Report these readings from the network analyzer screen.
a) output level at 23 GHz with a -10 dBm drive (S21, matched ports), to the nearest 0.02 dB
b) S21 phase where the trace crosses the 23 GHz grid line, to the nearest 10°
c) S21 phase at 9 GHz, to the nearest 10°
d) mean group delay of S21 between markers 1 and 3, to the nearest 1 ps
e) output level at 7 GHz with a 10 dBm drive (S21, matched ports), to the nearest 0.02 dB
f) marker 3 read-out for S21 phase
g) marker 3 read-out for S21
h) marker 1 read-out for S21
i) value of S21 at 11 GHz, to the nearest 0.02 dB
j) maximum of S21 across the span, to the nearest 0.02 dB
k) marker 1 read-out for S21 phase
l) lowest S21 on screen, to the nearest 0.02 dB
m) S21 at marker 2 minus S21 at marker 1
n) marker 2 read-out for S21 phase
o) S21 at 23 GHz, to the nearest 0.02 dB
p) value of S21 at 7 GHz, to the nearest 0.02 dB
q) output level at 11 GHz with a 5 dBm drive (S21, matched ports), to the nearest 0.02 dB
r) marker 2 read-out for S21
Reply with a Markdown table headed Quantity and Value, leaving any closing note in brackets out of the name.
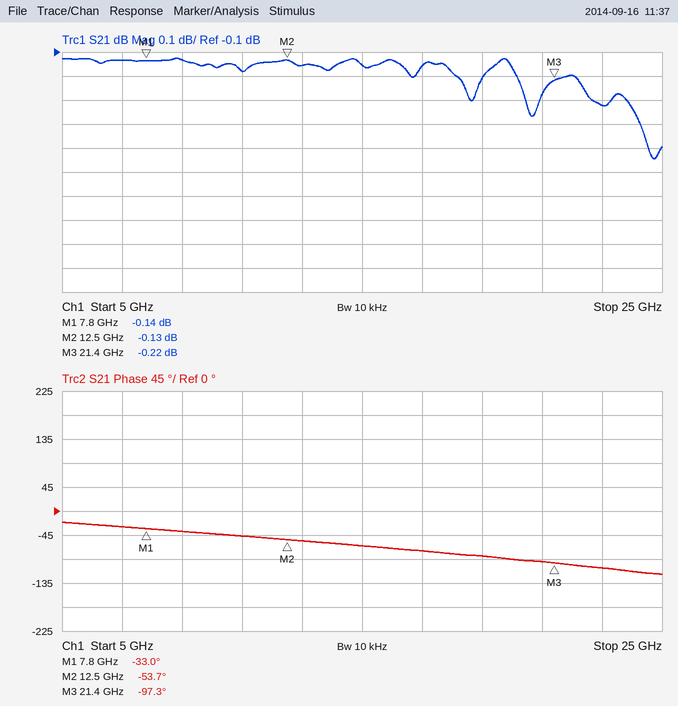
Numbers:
| Quantity | Value |
|---|---|
| output level at 23 GHz with a -10 dBm drive (S21, matched ports), to the nearest 0.02 dB | -10.32 dBm |
| S21 phase where the trace crosses the 23 GHz grid line, to the nearest 10° | -110° |
| S21 phase at 9 GHz, to the nearest 10° | -40° |
| mean group delay of S21 between markers 1 and 3, to the nearest 1 ps | 13 ps |
| output level at 7 GHz with a 10 dBm drive (S21, matched ports), to the nearest 0.02 dB | 9.86 dBm |
| marker 3 read-out for S21 phase | -97.3° |
| marker 3 read-out for S21 | -0.22 dB |
| marker 1 read-out for S21 | -0.14 dB |
| value of S21 at 11 GHz, to the nearest 0.02 dB | -0.18 dB |
| maximum of S21 across the span, to the nearest 0.02 dB | -0.12 dB |
| marker 1 read-out for S21 phase | -33.0° |
| lowest S21 on screen, to the nearest 0.02 dB | -0.54 dB |
| S21 at marker 2 minus S21 at marker 1 | 0.01 dB |
| marker 2 read-out for S21 phase | -53.7° |
| S21 at 23 GHz, to the nearest 0.02 dB | -0.32 dB |
| value of S21 at 7 GHz, to the nearest 0.02 dB | -0.14 dB |
| output level at 11 GHz with a 5 dBm drive (S21, matched ports), to the nearest 0.02 dB | 4.82 dBm |
| marker 2 read-out for S21 | -0.13 dB |
